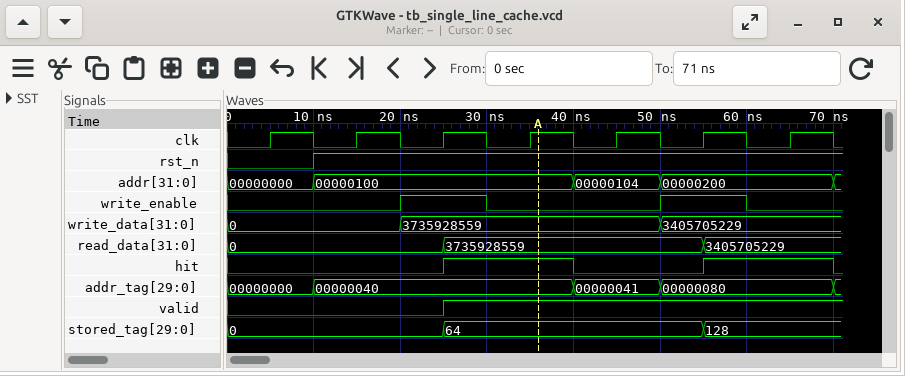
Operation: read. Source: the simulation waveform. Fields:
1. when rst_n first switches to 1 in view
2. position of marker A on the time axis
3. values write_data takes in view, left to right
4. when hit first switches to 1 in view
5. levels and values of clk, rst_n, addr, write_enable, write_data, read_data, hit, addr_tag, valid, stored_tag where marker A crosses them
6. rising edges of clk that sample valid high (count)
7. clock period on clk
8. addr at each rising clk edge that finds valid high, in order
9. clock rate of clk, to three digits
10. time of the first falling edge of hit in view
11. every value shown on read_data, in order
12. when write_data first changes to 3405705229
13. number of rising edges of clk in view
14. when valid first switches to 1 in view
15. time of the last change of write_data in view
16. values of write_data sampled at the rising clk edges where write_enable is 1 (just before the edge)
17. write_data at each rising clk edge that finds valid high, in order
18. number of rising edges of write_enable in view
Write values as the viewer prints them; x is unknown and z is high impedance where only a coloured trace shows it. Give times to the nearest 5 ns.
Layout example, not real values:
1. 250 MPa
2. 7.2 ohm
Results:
1. 10 ns
2. 35 ns
3. 0, 3735928559, 3405705229
4. 25 ns
5. clk=1, rst_n=1, addr=00000100, write_enable=0, write_data=3735928559, read_data=3735928559, hit=1, addr_tag=00000040, valid=1, stored_tag=64
6. 4
7. 10 ns
8. 00000100, 00000104, 00000200, 00000200
9. 100 MHz
10. 40 ns
11. 0, 3735928559, 3405705229
12. 50 ns
13. 7
14. 25 ns
15. 50 ns
16. 3735928559, 3405705229
17. 3735928559, 3735928559, 3405705229, 3405705229
18. 2
